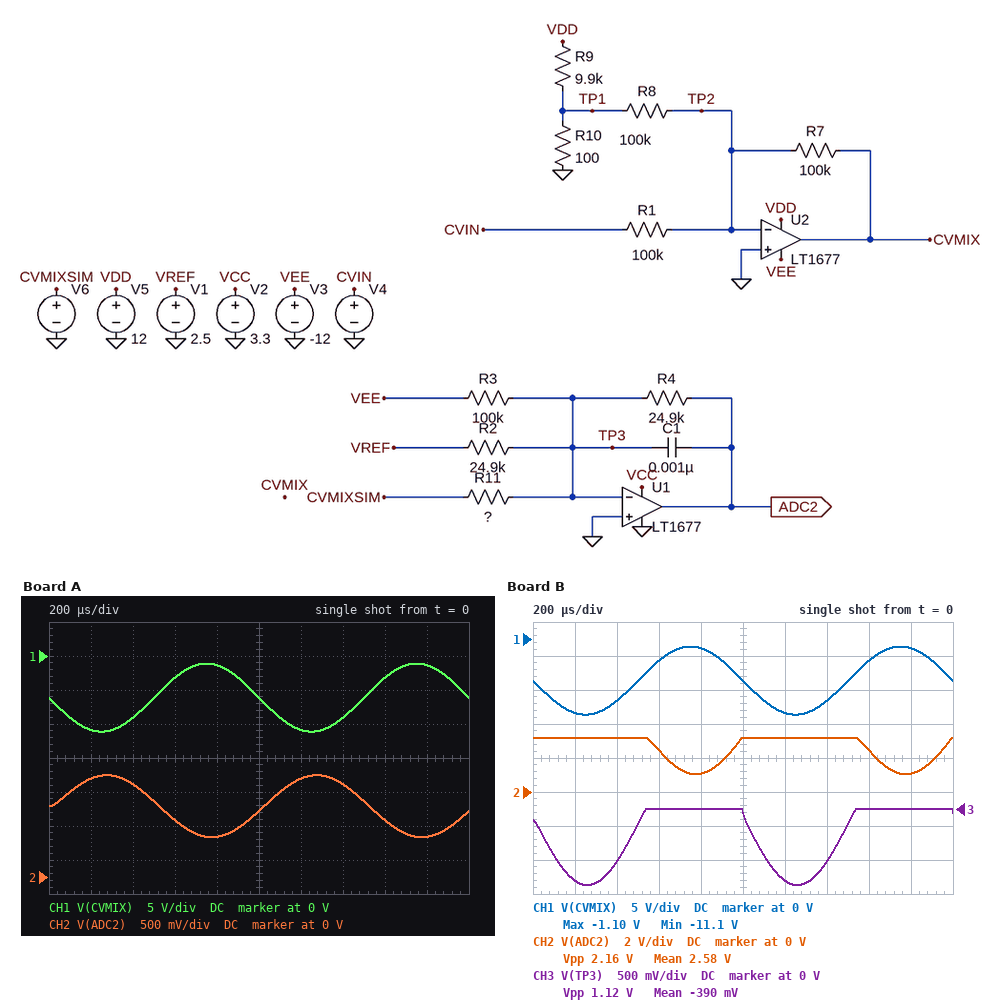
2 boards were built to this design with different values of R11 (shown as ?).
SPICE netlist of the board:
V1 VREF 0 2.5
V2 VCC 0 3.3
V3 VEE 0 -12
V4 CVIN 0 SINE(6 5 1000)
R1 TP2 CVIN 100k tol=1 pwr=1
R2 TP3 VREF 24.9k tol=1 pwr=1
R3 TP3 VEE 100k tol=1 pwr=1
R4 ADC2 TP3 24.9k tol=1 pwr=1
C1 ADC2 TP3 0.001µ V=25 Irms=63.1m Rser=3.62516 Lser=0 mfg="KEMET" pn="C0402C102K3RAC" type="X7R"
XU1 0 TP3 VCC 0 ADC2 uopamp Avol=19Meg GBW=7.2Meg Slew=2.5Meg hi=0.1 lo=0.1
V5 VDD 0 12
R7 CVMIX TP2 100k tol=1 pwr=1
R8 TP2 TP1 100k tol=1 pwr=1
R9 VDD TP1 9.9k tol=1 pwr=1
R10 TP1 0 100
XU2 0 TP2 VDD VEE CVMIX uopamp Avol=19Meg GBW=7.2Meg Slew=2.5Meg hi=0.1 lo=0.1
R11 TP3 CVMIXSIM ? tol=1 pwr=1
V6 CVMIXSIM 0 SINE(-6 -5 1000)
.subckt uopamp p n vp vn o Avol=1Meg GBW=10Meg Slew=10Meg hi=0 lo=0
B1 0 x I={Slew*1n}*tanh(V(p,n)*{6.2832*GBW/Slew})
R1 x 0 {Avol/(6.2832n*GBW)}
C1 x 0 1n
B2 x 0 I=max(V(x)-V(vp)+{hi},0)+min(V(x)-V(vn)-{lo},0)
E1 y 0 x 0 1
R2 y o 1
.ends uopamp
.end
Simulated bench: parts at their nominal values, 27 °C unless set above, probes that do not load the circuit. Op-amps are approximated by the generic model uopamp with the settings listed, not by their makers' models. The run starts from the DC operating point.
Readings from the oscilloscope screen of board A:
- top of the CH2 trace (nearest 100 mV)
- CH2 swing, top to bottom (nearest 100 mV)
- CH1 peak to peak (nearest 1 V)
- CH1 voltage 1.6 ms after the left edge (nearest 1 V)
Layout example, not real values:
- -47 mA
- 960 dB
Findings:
- 1.5 V
- 900 mV
- 10 V
- -3 V
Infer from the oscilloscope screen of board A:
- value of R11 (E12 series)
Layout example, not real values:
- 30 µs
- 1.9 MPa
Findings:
- 270 kΩ
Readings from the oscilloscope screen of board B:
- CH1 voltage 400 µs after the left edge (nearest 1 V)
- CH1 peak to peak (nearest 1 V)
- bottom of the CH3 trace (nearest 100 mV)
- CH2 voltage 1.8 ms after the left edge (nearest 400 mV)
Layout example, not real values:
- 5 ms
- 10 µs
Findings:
- -9 V
- 10 V
- -1.1 V
- 1.2 V
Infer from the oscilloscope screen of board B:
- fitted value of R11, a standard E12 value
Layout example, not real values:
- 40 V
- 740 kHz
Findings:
- 47 kΩ
